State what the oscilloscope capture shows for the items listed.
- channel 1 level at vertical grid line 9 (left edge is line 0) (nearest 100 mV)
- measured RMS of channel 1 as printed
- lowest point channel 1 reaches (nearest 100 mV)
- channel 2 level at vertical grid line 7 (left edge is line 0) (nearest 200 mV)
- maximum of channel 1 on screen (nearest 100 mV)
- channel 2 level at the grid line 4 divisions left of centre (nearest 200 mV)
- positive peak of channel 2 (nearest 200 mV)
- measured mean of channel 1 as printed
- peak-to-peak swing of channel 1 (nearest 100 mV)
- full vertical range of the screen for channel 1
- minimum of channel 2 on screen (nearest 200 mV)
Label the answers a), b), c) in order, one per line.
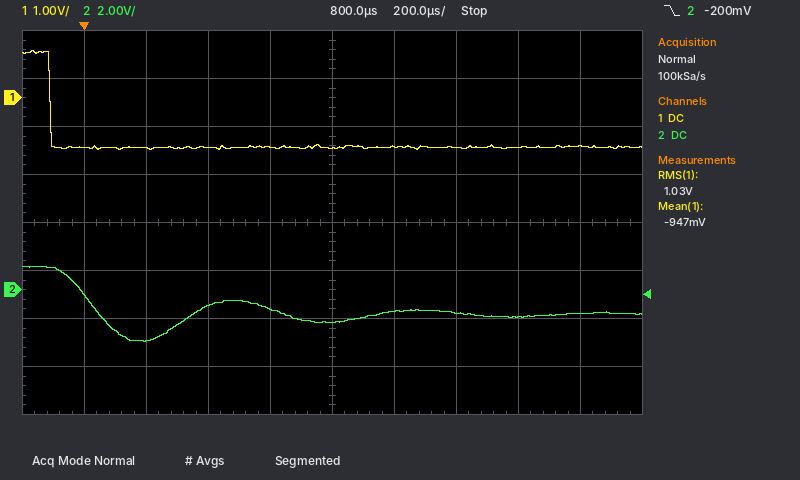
a) -1.0 V
b) 1.03 V
c) -1.1 V
d) -1.0 V
e) 1.0 V
f) -200 mV
g) 1.0 V
h) -947 mV
i) 2.1 V
j) 8 V
k) -2.2 V
